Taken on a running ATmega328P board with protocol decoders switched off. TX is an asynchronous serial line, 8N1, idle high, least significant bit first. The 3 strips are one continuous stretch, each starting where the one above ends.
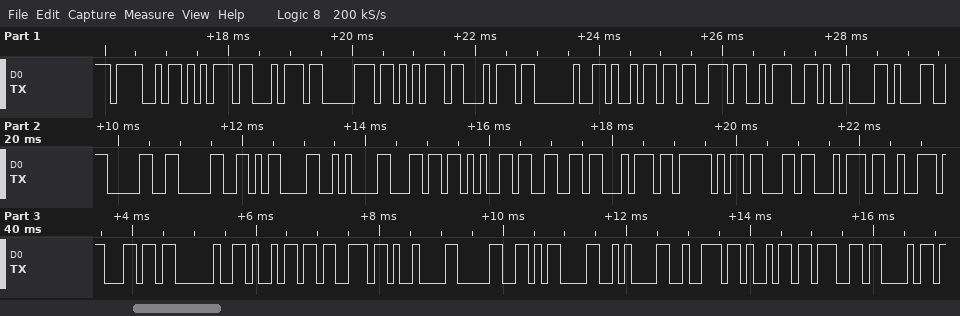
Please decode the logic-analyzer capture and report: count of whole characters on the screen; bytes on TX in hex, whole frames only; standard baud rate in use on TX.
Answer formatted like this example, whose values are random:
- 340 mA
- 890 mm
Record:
- 36
- 4F 75 74 70 75 74 20 69 73 3A 09 31 30 30 0D 0A 6C 65 66 74 5F 63 74 72 6C 20 69 73 09 30 0D 0A 72 69 67 68
- 9600 baud
